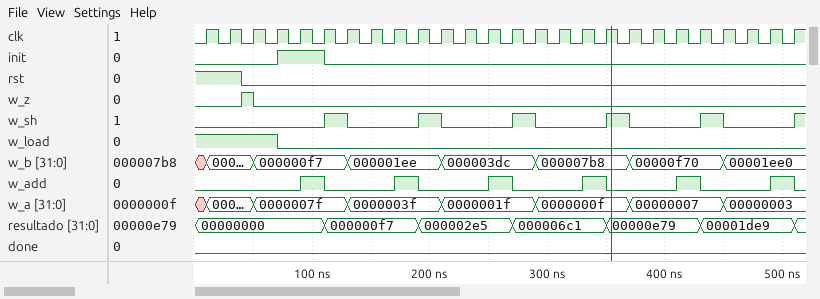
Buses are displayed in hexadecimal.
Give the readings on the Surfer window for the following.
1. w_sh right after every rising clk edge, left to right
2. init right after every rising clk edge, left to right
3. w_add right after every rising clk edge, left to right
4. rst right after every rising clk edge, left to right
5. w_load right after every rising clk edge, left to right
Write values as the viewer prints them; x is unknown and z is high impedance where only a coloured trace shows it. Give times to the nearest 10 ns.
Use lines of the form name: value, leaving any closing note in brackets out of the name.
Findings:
w_sh right after every rising clk edge, left to right: 0 0 0 0 0 1 0 0 0 1 0 0 0 1 0 0 0 1 0 0 0 1 0 0 0 1
init right after every rising clk edge, left to right: 0 0 0 1 1 0 0 0 0 0 0 0 0 0 0 0 0 0 0 0 0 0 0 0 0 0
w_add right after every rising clk edge, left to right: 0 0 0 0 1 0 0 0 1 0 0 0 1 0 0 0 1 0 0 0 1 0 0 0 1 0
rst right after every rising clk edge, left to right: 1 1 0 0 0 0 0 0 0 0 0 0 0 0 0 0 0 0 0 0 0 0 0 0 0 0
w_load right after every rising clk edge, left to right: 1 1 1 0 0 0 0 0 0 0 0 0 0 0 0 0 0 0 0 0 0 0 0 0 0 0
